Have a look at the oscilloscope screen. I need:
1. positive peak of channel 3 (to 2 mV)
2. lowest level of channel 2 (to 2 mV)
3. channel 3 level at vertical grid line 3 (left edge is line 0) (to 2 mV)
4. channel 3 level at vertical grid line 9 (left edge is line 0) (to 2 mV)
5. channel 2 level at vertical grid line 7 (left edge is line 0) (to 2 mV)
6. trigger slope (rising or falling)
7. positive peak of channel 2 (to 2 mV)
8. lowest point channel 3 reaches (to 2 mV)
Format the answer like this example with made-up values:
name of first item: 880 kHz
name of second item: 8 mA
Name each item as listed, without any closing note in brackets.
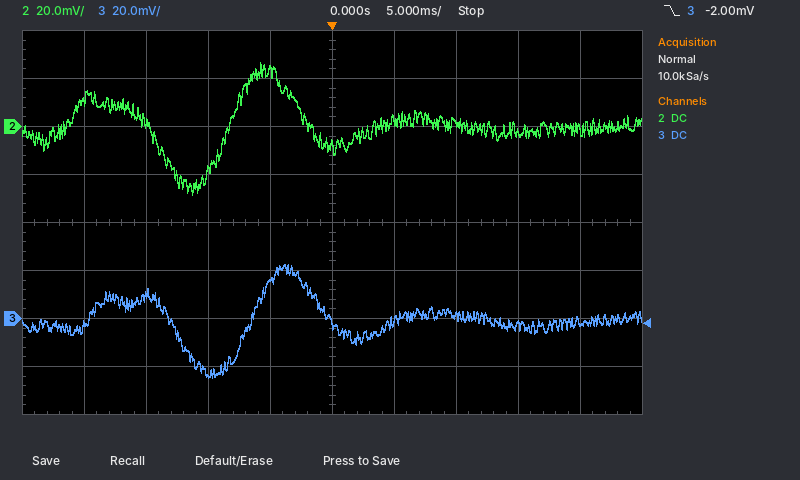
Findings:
positive peak of channel 3: 22 mV
lowest level of channel 2: -28 mV
channel 3 level at vertical grid line 3 (left edge is line 0): -22 mV
channel 3 level at vertical grid line 9 (left edge is line 0): -2 mV
channel 2 level at vertical grid line 7 (left edge is line 0): 2 mV
trigger slope: falling
positive peak of channel 2: 26 mV
lowest point channel 3 reaches: -24 mV
